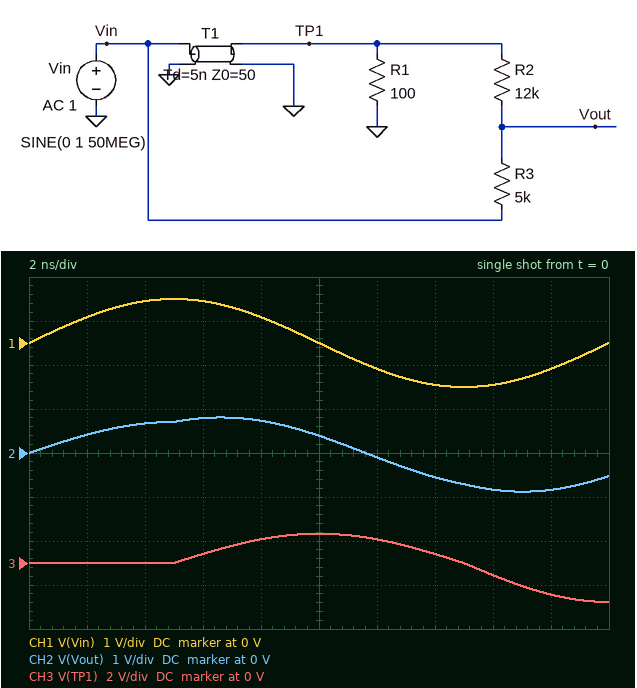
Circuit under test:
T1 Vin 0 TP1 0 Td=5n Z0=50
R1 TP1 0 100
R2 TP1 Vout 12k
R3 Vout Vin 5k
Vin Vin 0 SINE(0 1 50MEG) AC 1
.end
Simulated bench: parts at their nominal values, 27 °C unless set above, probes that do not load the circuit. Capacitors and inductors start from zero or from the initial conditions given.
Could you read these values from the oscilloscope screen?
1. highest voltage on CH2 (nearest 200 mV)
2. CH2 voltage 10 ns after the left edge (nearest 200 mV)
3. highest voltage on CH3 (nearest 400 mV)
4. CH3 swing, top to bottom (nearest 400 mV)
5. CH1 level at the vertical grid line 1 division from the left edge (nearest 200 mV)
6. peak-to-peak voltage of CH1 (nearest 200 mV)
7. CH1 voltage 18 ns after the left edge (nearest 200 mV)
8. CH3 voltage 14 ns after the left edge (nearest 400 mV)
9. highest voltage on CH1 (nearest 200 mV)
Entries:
800 mV
400 mV
1.2 V
3.2 V
600 mV
2.0 V
-600 mV
400 mV
1.0 V
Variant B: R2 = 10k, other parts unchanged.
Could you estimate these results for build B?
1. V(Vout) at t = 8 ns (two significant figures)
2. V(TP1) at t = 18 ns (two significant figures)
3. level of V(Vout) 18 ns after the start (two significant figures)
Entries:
750 mV
-1.4 V
-870 mV
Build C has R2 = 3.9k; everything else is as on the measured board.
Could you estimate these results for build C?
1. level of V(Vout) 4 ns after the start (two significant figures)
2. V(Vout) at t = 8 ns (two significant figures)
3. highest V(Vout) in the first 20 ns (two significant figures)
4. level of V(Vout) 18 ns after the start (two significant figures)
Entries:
420 mV
860 mV
870 mV
-1.1 V
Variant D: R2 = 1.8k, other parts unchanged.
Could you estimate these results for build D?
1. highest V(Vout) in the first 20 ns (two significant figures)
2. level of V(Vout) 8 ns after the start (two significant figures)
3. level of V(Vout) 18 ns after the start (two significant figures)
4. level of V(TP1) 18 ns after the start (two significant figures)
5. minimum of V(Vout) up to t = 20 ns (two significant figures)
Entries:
1.0 V
950 mV
-1.2 V
-1.4 V
-1.3 V
